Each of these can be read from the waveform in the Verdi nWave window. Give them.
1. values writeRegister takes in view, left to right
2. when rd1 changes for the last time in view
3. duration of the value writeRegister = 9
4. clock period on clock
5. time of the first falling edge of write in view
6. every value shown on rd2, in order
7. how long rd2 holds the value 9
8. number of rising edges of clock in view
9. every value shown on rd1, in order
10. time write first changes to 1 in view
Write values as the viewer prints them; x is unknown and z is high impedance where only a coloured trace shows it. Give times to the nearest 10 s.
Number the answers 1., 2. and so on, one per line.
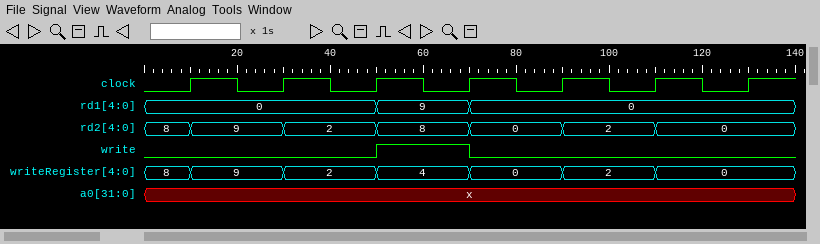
1. 8, 9, 2, 4, 0, 2, 0
2. 70 s
3. 20 s
4. 20 s
5. 70 s
6. 8, 9, 2, 8, 0, 2, 0
7. 20 s
8. 7
9. 0, 9, 0
10. 50 s
